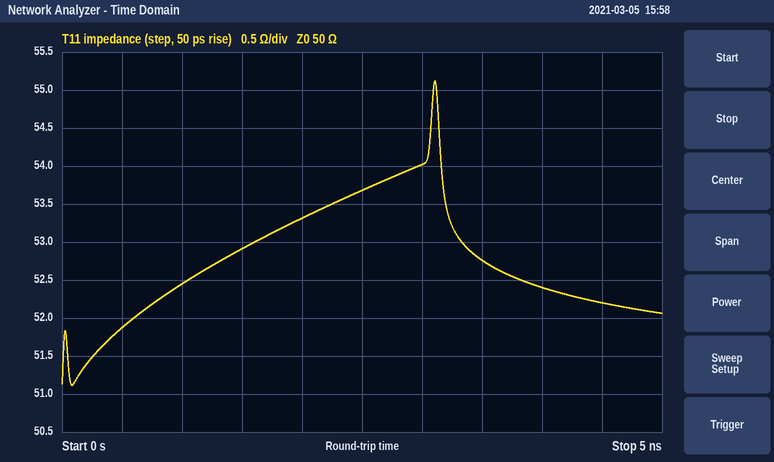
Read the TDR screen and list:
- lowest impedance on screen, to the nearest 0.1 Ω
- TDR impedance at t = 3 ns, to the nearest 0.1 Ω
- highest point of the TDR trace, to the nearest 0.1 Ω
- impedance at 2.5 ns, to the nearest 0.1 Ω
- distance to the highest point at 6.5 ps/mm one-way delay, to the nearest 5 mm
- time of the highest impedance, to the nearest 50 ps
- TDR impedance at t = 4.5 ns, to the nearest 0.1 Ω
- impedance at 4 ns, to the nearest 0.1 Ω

51.1 Ω
54.0 Ω
55.1 Ω
53.7 Ω
240 mm
3.10 ns
52.2 Ω
52.4 Ω
